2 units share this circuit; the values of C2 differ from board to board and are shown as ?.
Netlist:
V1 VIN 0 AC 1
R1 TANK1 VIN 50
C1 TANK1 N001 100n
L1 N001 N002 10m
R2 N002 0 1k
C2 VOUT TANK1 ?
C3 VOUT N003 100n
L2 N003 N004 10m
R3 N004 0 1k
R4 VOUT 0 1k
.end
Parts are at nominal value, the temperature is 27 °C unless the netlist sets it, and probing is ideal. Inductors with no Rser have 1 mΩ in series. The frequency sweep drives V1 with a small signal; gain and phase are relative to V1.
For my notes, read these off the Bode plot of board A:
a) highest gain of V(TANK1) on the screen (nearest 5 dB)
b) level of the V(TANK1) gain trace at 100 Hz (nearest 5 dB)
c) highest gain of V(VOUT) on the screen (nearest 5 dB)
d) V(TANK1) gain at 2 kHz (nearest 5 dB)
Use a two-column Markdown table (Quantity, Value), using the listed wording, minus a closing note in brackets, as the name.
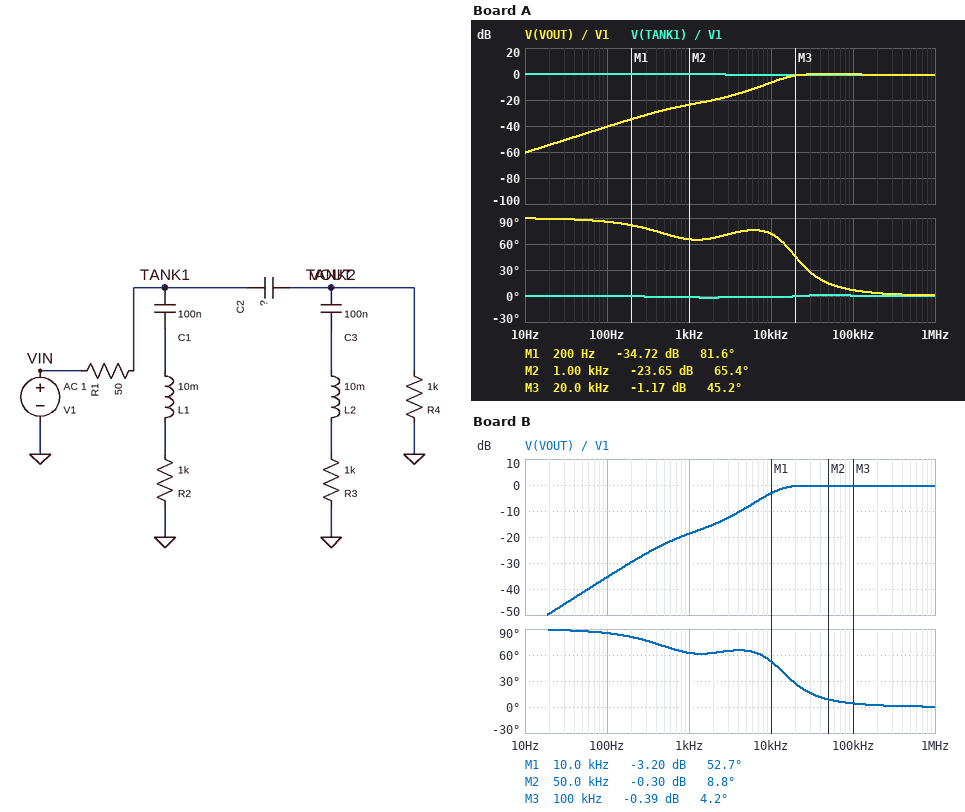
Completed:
| Quantity | Value |
|---|---|
| highest gain of V(TANK1) on the screen | 0 dB |
| level of the V(TANK1) gain trace at 100 Hz | 0 dB |
| highest gain of V(VOUT) on the screen | 0 dB |
| V(TANK1) gain at 2 kHz | 0 dB |
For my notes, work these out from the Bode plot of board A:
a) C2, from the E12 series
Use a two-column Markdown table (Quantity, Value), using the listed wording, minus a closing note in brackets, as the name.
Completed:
| Quantity | Value |
|---|---|
| C2, from the E12 series | 15 nF |
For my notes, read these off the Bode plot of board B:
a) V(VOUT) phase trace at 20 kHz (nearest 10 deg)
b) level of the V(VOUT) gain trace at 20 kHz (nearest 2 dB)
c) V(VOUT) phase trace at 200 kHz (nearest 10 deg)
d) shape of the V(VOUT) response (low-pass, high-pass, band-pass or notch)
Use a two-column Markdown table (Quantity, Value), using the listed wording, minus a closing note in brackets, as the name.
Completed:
| Quantity | Value |
|---|---|
| V(VOUT) phase trace at 20 kHz | 30 deg |
| level of the V(VOUT) gain trace at 20 kHz | 0 dB |
| V(VOUT) phase trace at 200 kHz | 0 deg |
| shape of the V(VOUT) response | high-pass |
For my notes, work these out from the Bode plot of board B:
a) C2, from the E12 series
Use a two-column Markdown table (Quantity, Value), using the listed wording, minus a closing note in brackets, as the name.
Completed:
| Quantity | Value |
|---|---|
| C2, from the E12 series | 27 nF |
